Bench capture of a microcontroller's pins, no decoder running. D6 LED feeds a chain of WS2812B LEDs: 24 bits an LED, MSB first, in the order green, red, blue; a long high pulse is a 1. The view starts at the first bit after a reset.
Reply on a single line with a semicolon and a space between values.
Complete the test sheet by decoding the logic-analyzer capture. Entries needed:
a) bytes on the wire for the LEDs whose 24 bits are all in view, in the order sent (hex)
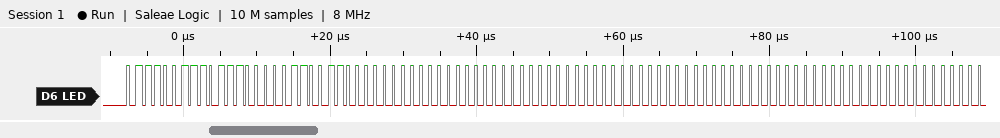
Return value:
73 B8 33 00 00 00 00 00 00
